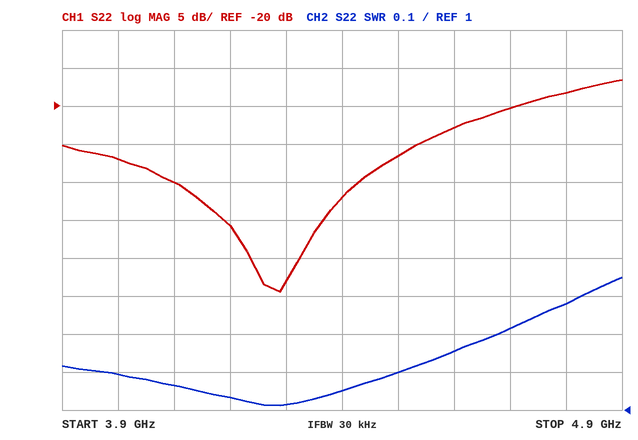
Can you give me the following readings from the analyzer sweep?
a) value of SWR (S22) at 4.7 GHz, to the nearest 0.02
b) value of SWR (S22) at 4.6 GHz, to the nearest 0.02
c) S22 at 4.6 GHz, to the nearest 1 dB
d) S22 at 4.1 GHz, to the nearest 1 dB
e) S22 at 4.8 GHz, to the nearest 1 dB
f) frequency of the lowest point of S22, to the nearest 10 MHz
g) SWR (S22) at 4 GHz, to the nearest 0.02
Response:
1.22
1.16
-23 dB
-30 dB
-18 dB
4.29 GHz
1.10
